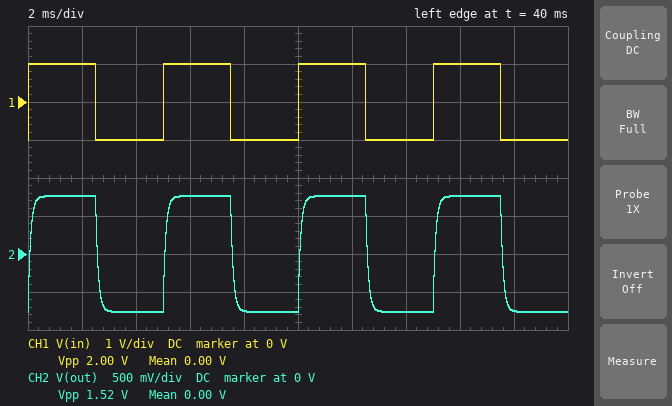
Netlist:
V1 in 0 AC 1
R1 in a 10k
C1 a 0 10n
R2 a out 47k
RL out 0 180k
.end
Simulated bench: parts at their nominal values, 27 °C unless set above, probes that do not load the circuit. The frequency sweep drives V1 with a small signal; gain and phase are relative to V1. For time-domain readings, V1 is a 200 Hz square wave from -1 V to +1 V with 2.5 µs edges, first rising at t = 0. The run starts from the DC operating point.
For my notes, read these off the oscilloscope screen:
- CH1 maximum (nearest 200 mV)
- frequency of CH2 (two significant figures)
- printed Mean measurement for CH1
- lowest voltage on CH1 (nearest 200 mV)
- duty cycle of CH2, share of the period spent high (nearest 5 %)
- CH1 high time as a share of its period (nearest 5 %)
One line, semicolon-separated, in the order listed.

1.0 V; 200 Hz; 0.00 V; -1.0 V; 50 %; 50 %
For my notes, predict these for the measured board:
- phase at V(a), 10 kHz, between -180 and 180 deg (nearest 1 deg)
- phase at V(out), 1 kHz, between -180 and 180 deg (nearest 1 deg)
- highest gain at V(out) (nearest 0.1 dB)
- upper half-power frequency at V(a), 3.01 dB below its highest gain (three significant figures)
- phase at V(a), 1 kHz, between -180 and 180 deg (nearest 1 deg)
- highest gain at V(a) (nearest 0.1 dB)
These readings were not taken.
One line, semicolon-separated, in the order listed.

-81 deg; -31 deg; -2.4 dB; 1.66 kHz; -31 deg; -0.4 dB
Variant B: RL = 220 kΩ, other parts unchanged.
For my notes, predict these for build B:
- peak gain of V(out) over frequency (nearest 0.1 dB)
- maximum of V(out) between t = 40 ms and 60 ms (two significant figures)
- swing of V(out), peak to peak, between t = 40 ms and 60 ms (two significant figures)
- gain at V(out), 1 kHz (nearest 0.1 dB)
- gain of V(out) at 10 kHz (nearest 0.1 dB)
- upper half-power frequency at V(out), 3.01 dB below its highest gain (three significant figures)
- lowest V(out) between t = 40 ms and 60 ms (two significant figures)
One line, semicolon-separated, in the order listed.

-2.0 dB; 790 mV; 1.6 V; -3.4 dB; -17.8 dB; 1.65 kHz; -790 mV
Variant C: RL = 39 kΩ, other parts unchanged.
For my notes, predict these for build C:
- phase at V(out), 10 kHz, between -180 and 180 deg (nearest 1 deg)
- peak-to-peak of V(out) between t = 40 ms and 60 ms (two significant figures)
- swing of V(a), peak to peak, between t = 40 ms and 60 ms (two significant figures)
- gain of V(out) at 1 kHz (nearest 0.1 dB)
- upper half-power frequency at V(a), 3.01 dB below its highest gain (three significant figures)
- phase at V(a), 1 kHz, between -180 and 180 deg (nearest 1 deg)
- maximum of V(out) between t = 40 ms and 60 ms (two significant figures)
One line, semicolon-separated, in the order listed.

-80 deg; 810 mV; 1.8 V; -9.0 dB; 1.78 kHz; -29 deg; 410 mV
